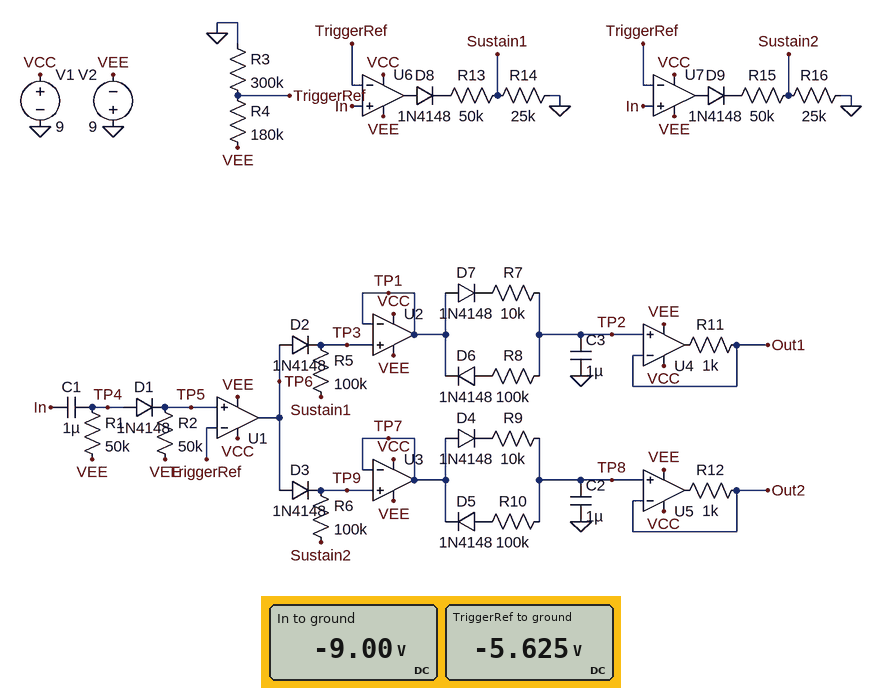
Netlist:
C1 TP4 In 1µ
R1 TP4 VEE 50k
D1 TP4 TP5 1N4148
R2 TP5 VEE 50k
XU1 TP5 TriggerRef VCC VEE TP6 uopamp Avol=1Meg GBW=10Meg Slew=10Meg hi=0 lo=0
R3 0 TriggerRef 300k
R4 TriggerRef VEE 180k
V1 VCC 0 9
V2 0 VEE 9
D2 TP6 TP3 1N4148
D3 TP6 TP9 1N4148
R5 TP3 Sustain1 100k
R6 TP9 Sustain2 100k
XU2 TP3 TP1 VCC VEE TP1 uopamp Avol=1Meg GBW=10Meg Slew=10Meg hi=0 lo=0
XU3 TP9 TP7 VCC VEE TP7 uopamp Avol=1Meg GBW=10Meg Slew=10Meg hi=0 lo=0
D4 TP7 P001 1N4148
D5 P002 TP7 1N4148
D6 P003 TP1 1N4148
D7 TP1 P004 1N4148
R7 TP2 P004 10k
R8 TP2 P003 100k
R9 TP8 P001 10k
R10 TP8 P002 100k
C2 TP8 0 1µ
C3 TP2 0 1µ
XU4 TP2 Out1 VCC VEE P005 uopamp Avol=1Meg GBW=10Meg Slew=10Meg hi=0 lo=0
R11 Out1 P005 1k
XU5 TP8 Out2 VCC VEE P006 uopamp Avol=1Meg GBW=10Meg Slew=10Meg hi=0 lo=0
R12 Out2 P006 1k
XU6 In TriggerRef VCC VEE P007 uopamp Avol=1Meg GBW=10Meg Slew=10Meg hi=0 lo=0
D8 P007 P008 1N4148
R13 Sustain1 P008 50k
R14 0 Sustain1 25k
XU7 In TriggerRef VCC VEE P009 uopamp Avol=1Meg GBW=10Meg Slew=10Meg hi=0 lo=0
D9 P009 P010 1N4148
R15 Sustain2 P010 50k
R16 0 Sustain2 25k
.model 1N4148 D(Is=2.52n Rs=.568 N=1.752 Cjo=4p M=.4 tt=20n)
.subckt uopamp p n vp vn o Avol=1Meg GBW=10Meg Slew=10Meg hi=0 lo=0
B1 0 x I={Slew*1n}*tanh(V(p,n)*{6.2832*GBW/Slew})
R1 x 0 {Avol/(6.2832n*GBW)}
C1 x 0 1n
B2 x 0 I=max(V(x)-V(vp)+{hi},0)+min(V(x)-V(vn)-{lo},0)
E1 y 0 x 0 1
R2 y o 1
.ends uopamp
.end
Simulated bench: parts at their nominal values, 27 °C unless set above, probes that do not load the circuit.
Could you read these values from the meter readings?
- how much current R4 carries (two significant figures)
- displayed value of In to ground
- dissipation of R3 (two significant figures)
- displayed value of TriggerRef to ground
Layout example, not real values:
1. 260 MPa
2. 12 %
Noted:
1. 19 µA
2. -9.00 V
3. 110 µW
4. -5.625 V
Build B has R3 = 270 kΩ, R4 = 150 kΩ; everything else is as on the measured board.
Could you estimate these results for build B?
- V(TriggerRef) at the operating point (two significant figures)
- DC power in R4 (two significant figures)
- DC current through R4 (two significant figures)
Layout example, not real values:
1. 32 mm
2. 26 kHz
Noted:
1. -5.8 V
2. 69 µW
3. 21 µA
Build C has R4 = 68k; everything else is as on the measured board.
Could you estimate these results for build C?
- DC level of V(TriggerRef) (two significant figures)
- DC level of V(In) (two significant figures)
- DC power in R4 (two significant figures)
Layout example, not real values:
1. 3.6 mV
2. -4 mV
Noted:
1. -7.3 V
2. -9.0 V
3. 41 µW
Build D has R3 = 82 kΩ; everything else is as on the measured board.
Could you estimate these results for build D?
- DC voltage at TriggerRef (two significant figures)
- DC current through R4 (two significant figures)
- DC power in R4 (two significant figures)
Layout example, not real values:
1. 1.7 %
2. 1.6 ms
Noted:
1. -2.8 V
2. 34 µA
3. 210 µW
